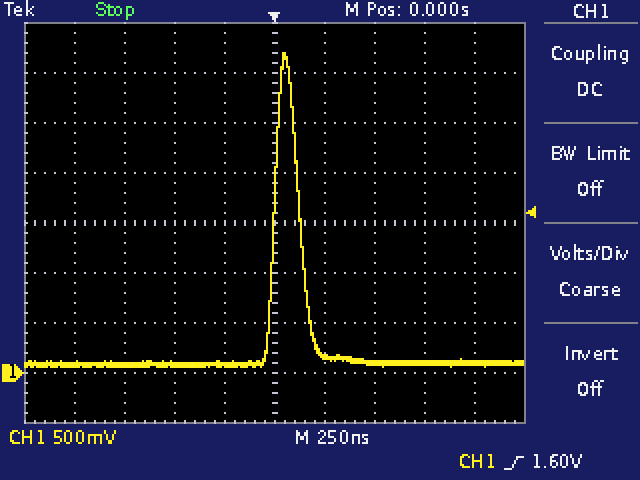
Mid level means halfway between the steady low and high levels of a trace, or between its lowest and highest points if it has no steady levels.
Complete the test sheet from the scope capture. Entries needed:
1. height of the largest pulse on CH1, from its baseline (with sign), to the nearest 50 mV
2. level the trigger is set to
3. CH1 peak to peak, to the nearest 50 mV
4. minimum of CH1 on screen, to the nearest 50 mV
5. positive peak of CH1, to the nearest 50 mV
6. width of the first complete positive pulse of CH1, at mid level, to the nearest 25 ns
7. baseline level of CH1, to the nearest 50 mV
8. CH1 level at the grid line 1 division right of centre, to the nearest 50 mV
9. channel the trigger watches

+3.10 V
1.60 V
3.15 V
50 mV
3.20 V
125 ns
100 mV
150 mV
CH1
